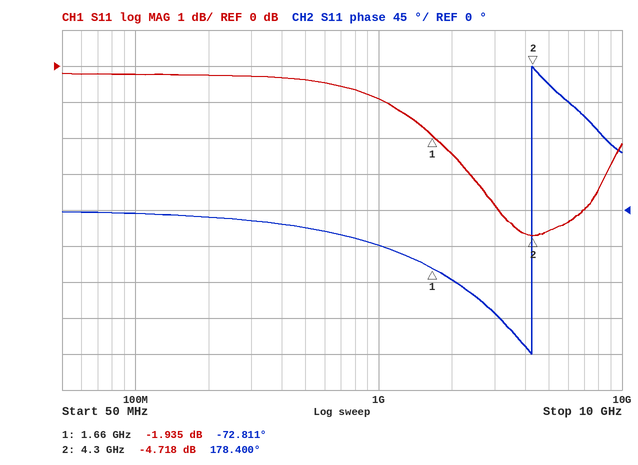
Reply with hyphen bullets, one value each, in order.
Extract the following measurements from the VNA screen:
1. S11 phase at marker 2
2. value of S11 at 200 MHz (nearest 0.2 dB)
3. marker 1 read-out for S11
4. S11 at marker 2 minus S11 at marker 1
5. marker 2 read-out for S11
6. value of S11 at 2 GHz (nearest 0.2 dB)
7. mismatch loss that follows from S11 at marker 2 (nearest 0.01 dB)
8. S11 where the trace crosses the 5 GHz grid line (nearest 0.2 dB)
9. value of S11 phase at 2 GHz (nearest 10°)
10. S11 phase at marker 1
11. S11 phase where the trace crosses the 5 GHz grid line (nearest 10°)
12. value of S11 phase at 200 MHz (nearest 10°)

- 178.400°
- -0.2 dB
- -1.935 dB
- -2.783 dB
- -4.718 dB
- -2.4 dB
- 1.79 dB
- -4.6 dB
- -90°
- -72.811°
- 160°
- -10°
